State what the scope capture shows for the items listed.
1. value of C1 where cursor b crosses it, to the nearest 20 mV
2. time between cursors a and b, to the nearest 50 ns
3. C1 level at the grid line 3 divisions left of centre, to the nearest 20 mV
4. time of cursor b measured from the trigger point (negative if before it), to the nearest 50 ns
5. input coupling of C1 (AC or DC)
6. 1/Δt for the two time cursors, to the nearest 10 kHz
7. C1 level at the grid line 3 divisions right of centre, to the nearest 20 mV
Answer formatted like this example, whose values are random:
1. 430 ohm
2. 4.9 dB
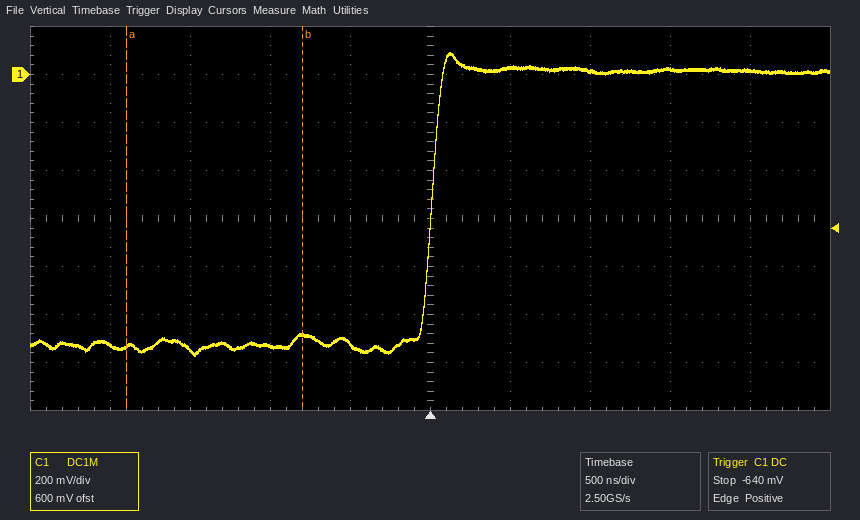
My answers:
1. -1.08 V
2. 1.10 µs
3. -1.14 V
4. -800 ns
5. DC
6. 910 kHz
7. 20 mV
